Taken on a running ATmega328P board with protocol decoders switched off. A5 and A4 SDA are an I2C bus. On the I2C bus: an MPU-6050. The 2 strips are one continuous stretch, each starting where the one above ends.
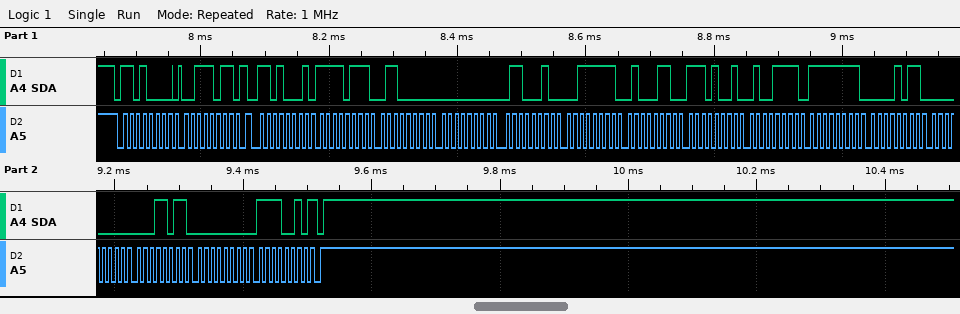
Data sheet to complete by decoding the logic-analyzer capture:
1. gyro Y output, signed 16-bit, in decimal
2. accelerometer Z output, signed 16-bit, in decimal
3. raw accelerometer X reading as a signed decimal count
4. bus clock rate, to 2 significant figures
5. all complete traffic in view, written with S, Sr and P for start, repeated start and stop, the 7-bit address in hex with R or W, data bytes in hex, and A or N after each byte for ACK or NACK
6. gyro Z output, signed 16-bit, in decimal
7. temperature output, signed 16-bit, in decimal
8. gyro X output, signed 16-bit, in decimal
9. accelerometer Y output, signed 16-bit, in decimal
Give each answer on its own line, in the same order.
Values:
27
16198
-2208
100 kHz
S 68W A 3B A Sr 68R A F7 A 60 A 00 A 62 A 3F A 46 A E9 A 4F A FF A 0B A 00 A 1B A 00 A F2 N P
242
-5809
-245
98
